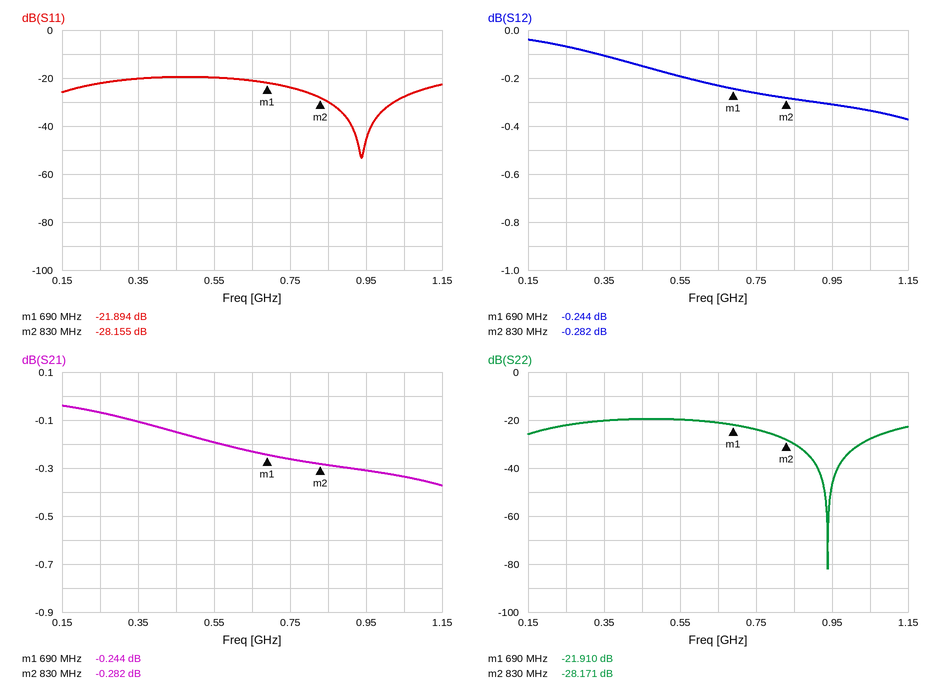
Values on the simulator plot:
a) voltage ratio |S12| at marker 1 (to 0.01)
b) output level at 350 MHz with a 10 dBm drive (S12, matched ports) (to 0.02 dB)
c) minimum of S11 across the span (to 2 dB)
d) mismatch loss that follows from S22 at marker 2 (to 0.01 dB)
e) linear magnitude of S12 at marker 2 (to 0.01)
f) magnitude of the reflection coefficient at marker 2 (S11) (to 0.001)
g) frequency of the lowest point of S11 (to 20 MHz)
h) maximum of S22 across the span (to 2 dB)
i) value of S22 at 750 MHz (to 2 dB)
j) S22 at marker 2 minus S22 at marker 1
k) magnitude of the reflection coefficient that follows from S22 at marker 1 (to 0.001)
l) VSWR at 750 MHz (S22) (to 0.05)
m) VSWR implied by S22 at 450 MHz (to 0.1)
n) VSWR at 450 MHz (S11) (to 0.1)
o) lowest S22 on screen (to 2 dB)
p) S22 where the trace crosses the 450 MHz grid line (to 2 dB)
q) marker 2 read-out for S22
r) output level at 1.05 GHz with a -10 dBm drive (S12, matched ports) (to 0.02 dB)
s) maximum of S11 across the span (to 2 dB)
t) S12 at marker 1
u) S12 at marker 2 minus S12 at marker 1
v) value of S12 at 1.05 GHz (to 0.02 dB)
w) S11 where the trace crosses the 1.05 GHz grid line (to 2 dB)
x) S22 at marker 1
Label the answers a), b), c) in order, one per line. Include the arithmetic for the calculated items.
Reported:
a) 10^(-0.244/20) ≈ 0.97
b) 10 dBm + (-0.10 dB) = 9.90 dBm
c) -54 dB
d) −10 log10(1 − 10^(-28.171/10)) ≈ 0.01 dB
e) 10^(-0.282/20) ≈ 0.97
f) 10^(-28.155/20) ≈ 0.039
g) 940 MHz
h) -20 dB
i) -24 dB
j) -28.171 − (-21.91) = -6.261 dB
k) 10^(-21.91/20) ≈ 0.080
l) |Γ| = 10^(-24/20) = 0.0631; VSWR = (1 + 0.0631)/(1 − 0.0631) ≈ 1.13, so 1.15 to the nearest 0.05
m) |Γ| = 10^(-20/20) = 0.1000; VSWR = (1 + 0.1000)/(1 − 0.1000) ≈ 1.2
n) |Γ| = 10^(-20/20) = 0.1000; VSWR = (1 + 0.1000)/(1 − 0.1000) ≈ 1.2
o) -82 dB
p) -20 dB
q) -28.171 dB
r) -10 dBm + (-0.34 dB) = -10.34 dBm
s) -20 dB
t) -0.244 dB
u) -0.282 − (-0.244) = -0.038 dB
v) -0.34 dB
w) -28 dB
x) -21.910 dB
